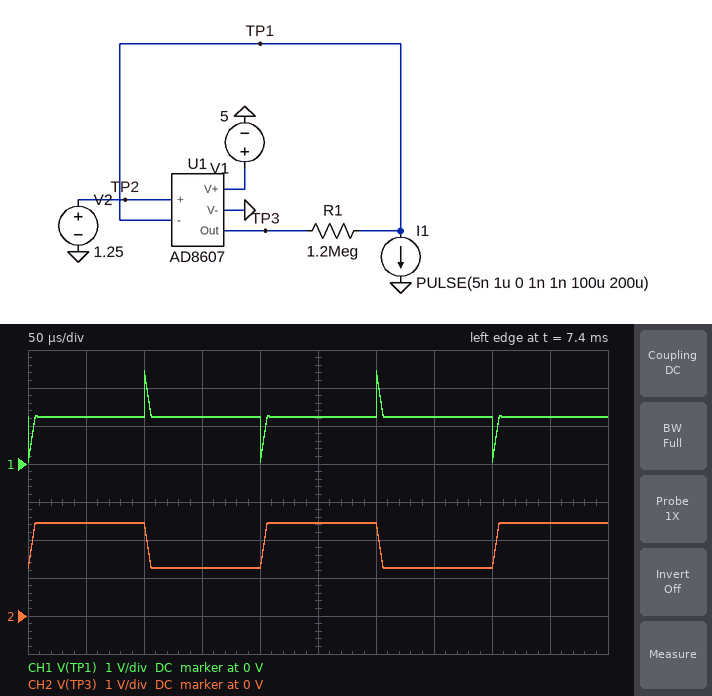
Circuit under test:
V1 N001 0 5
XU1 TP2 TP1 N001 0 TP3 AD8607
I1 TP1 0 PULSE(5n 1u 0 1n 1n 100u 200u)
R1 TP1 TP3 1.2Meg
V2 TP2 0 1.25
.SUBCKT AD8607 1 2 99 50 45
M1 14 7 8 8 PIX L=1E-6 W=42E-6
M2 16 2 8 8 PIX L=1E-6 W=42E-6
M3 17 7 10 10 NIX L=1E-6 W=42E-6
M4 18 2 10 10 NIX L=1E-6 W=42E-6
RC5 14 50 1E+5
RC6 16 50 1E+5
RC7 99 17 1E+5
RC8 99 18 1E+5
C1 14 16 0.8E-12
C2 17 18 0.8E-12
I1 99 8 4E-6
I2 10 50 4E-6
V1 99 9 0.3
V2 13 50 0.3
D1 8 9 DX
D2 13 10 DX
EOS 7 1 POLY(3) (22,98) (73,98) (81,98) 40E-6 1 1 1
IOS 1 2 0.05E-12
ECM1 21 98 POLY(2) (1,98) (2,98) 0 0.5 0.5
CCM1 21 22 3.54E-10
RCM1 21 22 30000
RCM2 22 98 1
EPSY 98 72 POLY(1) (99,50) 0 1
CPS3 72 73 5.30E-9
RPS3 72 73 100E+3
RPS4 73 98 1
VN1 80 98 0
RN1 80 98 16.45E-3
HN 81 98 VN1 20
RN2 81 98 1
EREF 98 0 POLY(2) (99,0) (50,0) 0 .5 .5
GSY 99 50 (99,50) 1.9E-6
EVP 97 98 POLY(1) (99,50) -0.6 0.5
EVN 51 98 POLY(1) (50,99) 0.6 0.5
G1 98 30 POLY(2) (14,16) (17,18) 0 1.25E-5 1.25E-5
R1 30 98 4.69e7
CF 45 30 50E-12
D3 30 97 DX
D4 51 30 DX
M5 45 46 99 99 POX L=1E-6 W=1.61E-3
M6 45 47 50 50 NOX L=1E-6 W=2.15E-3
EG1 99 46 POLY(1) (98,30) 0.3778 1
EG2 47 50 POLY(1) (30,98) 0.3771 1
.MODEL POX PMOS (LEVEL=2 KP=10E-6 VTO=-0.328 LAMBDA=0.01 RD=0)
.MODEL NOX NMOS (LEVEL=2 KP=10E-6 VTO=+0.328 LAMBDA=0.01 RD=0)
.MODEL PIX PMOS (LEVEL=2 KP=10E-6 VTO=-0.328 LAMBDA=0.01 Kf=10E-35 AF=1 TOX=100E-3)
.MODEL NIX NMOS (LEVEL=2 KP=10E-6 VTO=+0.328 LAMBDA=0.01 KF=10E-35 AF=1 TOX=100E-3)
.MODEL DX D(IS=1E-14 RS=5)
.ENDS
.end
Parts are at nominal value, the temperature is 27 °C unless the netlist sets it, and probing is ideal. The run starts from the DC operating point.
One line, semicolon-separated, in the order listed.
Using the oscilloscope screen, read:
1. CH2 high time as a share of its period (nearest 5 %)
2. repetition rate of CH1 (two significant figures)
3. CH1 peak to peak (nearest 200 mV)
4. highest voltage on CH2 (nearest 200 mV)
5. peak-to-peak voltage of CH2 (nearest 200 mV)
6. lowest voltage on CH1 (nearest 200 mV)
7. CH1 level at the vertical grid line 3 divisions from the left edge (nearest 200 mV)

50 %; 5.0 kHz; 2.4 V; 2.4 V; 1.2 V; 0 V; 1.2 V
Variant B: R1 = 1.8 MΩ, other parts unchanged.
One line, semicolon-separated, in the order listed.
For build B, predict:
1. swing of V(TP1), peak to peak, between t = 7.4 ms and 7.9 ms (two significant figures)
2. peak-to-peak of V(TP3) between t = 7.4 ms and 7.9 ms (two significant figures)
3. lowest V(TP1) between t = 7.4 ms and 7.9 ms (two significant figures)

3.6 V; 1.8 V; -540 mV
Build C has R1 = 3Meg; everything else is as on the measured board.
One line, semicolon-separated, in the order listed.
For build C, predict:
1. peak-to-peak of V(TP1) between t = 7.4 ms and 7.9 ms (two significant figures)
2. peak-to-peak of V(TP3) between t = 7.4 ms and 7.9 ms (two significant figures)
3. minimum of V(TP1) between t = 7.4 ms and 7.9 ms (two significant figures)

6.0 V; 3.0 V; -1.7 V
